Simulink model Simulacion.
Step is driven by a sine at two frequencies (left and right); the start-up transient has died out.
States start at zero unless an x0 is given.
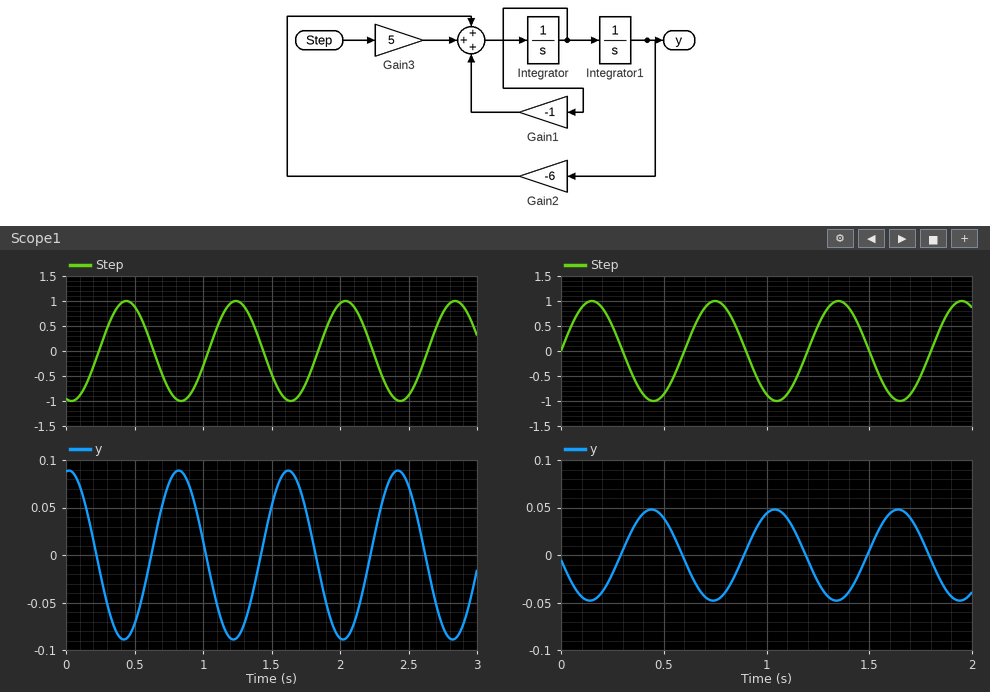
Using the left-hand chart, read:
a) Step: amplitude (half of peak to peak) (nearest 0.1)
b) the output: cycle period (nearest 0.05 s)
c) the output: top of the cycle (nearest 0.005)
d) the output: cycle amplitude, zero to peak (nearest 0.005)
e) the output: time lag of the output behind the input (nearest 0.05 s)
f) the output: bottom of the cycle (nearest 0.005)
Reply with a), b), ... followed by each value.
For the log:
a) 1.0
b) 0.80 s
c) 0.090
d) 0.090
e) 0.40 s
f) -0.090
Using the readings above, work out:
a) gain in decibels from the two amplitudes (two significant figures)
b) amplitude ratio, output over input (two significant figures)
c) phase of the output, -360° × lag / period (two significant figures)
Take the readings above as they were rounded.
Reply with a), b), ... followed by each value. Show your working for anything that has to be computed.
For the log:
a) 20 log10(0.09 / 1) = -21 dB
b) 0.09 / 1 = 0.090
c) -360 × 0.4 / 0.8 = -180°
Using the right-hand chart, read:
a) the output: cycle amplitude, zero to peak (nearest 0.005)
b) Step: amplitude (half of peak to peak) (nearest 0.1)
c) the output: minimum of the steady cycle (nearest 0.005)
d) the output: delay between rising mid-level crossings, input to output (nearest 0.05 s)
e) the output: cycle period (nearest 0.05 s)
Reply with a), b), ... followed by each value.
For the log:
a) 0.050
b) 1.0
c) -0.050
d) 0.30 s
e) 0.60 s
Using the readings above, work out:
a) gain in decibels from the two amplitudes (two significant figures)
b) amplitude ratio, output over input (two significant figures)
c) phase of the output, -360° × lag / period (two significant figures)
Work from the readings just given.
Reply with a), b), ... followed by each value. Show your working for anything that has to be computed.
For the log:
a) 20 log10(0.05 / 1) = -26 dB
b) 0.05 / 1 = 0.050
c) -360 × 0.3 / 0.6 = -180°
